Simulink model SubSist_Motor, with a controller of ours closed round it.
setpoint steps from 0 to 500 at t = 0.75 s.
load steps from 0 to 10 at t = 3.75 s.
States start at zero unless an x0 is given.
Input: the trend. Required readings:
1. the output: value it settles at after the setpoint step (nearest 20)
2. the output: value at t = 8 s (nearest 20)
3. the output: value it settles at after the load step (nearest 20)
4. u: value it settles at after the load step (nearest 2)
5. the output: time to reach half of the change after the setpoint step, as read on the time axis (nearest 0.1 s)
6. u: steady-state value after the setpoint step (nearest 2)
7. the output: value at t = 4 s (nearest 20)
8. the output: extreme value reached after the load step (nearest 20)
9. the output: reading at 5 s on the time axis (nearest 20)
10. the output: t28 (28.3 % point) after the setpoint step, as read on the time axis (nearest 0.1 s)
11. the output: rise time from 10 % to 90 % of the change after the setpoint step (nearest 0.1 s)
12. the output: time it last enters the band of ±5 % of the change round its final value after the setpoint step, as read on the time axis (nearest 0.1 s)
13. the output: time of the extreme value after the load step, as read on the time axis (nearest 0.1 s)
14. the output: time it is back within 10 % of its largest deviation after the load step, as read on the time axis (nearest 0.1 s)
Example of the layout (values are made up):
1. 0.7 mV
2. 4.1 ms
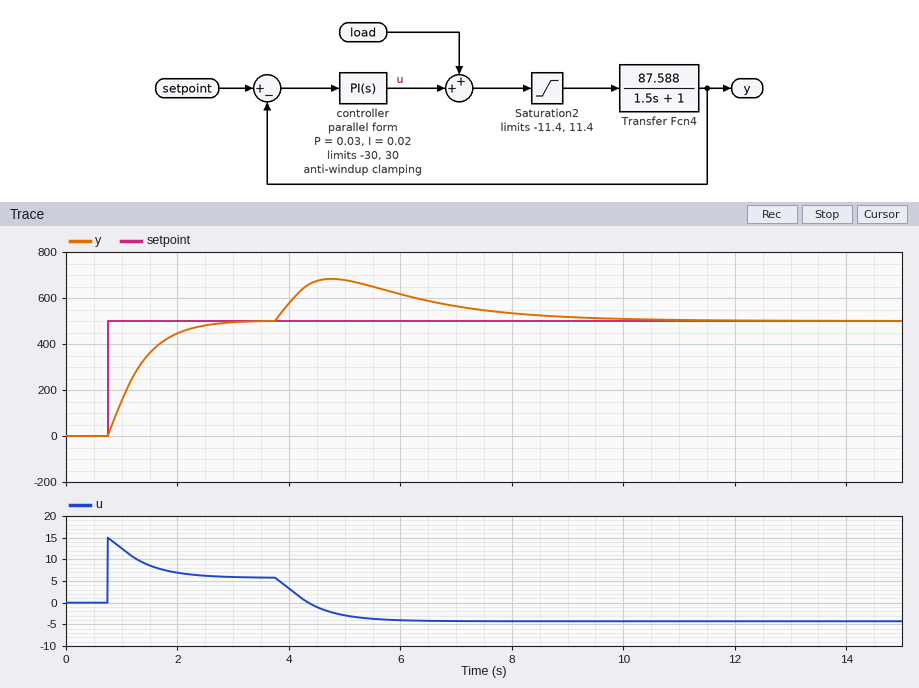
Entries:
1. 500
2. 540
3. 500
4. -4
5. 1.2 s
6. 6
7. 580
8. 680
9. 680
10. 1.0 s
11. 1.2 s
12. 2.4 s
13. 4.8 s
14. 8.9 s
